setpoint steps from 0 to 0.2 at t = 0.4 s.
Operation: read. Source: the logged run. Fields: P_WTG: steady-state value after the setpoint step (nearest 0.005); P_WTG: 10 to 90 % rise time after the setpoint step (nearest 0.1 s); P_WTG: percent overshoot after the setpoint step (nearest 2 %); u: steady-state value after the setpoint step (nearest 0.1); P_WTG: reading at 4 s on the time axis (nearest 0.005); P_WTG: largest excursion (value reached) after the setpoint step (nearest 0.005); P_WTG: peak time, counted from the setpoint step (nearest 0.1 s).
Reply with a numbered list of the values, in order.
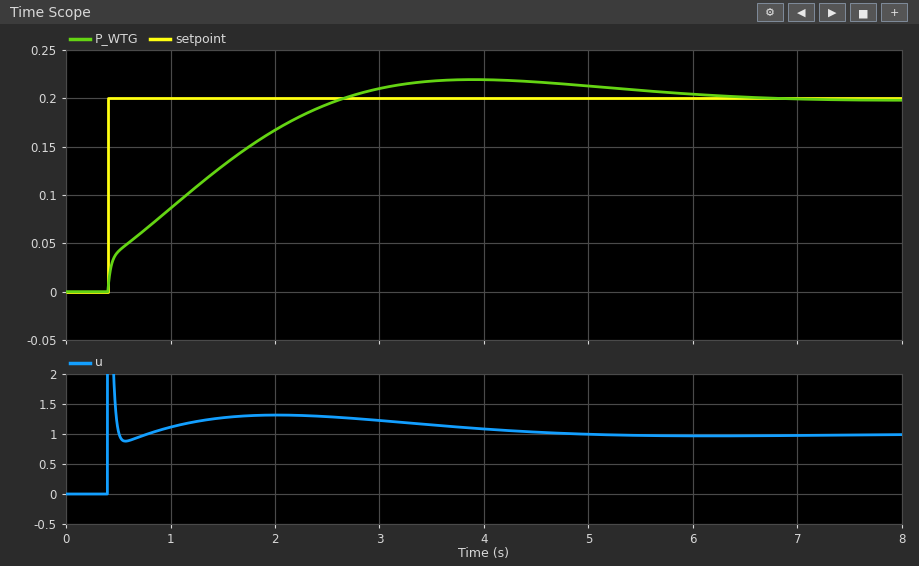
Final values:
1. 0.200
2. 1.8 s
3. 10 %
4. 1.0
5. 0.220
6. 0.220
7. 3.5 s
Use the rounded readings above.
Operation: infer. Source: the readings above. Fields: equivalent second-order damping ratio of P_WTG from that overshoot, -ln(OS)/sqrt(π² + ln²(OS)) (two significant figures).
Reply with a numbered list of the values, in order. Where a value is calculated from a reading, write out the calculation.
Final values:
1. ln(0.1) = -2.303; 2.303 / sqrt(9.870 + 5.302) = 0.59
